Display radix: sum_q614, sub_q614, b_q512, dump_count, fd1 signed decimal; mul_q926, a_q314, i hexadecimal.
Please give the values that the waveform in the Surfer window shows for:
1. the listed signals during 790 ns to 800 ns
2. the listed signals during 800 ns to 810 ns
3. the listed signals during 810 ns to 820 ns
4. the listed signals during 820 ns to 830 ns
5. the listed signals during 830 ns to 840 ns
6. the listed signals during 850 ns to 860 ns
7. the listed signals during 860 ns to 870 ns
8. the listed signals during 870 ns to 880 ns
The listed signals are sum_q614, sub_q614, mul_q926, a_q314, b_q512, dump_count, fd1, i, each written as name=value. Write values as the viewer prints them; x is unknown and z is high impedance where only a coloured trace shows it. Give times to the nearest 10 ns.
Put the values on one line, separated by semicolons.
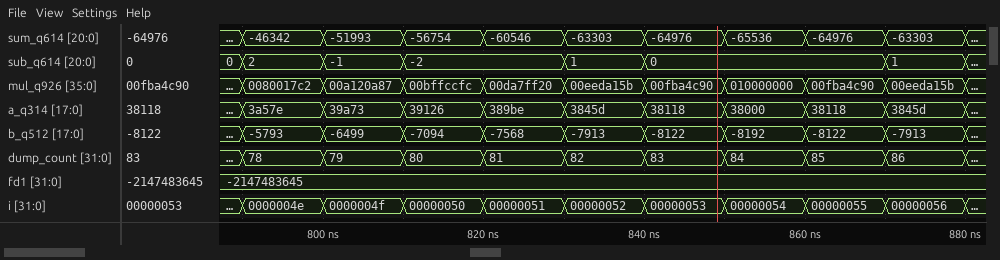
sum_q614=-46342, sub_q614=2, mul_q926=0080017c2, a_q314=3a57e, b_q512=-5793, dump_count=78, fd1=-2147483645, i=0000004e; sum_q614=-51993, sub_q614=-1, mul_q926=00a120a87, a_q314=39a73, b_q512=-6499, dump_count=79, fd1=-2147483645, i=0000004f; sum_q614=-56754, sub_q614=-2, mul_q926=00bffccfc, a_q314=39126, b_q512=-7094, dump_count=80, fd1=-2147483645, i=00000050; sum_q614=-60546, sub_q614=-2, mul_q926=00da7ff20, a_q314=389be, b_q512=-7568, dump_count=81, fd1=-2147483645, i=00000051; sum_q614=-63303, sub_q614=1, mul_q926=00eeda15b, a_q314=3845d, b_q512=-7913, dump_count=82, fd1=-2147483645, i=00000052; sum_q614=-65536, sub_q614=0, mul_q926=010000000, a_q314=38000, b_q512=-8192, dump_count=84, fd1=-2147483645, i=00000054; sum_q614=-64976, sub_q614=0, mul_q926=00fba4c90, a_q314=38118, b_q512=-8122, dump_count=85, fd1=-2147483645, i=00000055; sum_q614=-63303, sub_q614=1, mul_q926=00eeda15b, a_q314=3845d, b_q512=-7913, dump_count=86, fd1=-2147483645, i=00000056
